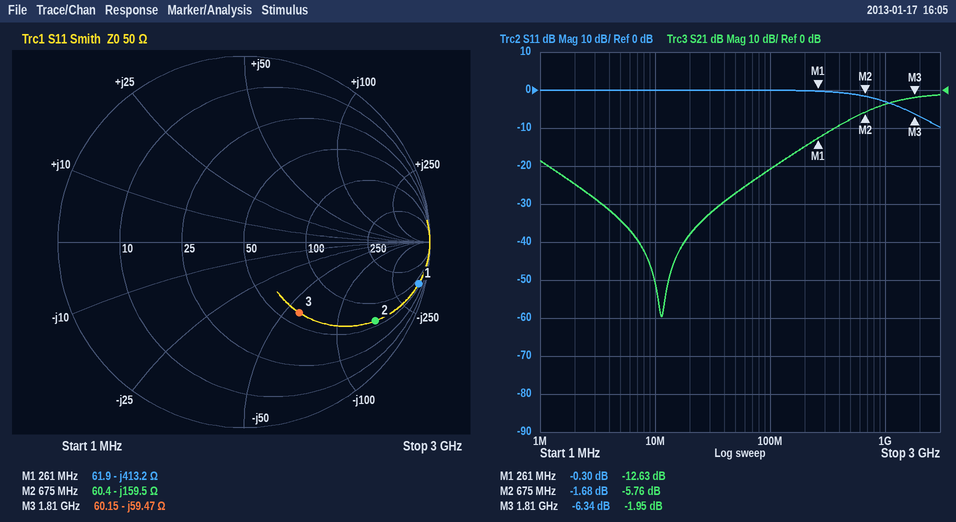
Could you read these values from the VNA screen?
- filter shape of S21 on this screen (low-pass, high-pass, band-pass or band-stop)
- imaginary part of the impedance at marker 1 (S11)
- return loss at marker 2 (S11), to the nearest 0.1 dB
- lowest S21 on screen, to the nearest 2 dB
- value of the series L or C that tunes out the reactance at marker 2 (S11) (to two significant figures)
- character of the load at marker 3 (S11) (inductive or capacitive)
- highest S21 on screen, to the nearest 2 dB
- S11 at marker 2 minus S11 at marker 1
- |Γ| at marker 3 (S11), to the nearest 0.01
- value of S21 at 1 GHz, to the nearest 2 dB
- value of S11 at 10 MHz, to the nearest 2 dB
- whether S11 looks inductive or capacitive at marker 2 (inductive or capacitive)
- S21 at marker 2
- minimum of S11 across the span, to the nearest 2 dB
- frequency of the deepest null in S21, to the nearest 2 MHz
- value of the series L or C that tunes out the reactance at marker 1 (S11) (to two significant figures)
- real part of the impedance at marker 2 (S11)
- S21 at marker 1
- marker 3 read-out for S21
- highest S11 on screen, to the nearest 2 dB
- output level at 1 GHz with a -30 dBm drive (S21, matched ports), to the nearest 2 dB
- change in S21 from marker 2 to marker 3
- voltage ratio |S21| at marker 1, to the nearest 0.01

high-pass
-413.2 Ω
1.7 dB
-60 dB
38 nH
capacitive
-2 dB
-1.38 dB
0.48
-4 dB
0 dB
capacitive
-5.76 dB
-10 dB
12 MHz
250 nH
60.4 Ω
-12.63 dB
-1.95 dB
0 dB
-34 dBm
3.81 dB
0.23
